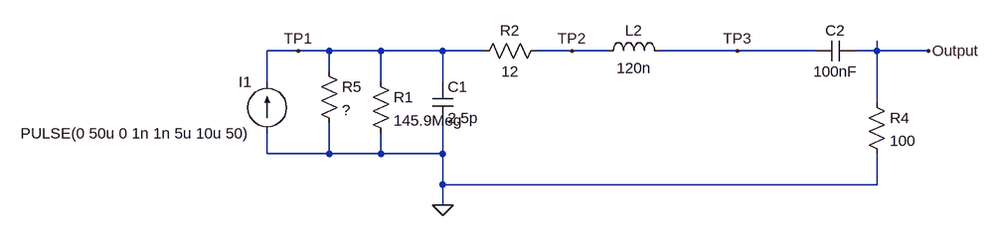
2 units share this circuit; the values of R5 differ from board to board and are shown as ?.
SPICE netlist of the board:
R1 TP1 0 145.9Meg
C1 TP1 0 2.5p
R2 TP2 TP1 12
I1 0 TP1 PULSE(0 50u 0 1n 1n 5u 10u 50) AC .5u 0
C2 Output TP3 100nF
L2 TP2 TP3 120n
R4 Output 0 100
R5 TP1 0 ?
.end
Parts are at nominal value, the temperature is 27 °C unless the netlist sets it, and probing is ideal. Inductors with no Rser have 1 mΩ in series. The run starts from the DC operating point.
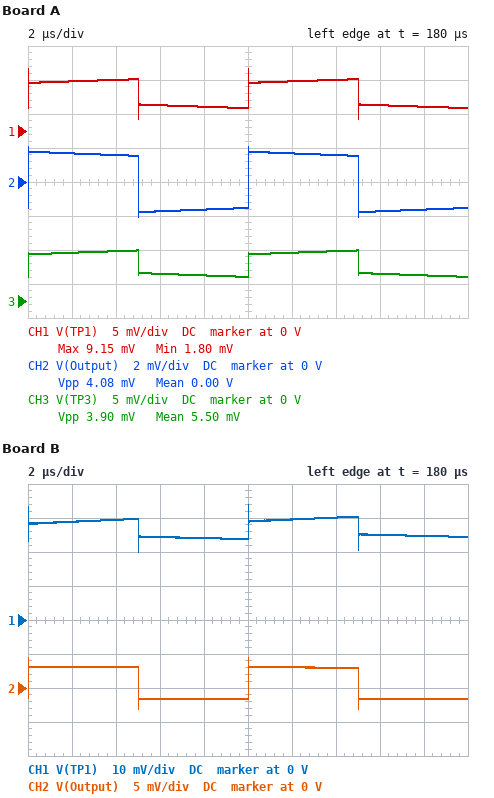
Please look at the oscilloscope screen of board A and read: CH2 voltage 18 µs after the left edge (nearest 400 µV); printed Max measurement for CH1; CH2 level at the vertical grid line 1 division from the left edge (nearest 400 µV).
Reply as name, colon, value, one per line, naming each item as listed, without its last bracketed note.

CH2 voltage 18 µs after the left edge: -1.6 mV
printed Max measurement for CH1: 9.15 mV
CH2 level at the vertical grid line 1 division from the left edge: 1.6 mV
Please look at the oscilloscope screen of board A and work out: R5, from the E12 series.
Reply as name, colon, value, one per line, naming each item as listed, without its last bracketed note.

R5, from the E12 series: 220 Ω
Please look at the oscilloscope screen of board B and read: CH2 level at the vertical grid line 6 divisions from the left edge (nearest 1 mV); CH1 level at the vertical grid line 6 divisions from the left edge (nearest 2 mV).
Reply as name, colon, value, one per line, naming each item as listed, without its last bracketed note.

CH2 level at the vertical grid line 6 divisions from the left edge: 3 mV
CH1 level at the vertical grid line 6 divisions from the left edge: 30 mV
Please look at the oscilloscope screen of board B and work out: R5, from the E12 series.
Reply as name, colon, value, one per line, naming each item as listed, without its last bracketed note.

R5, from the E12 series: 1.5 kΩ
